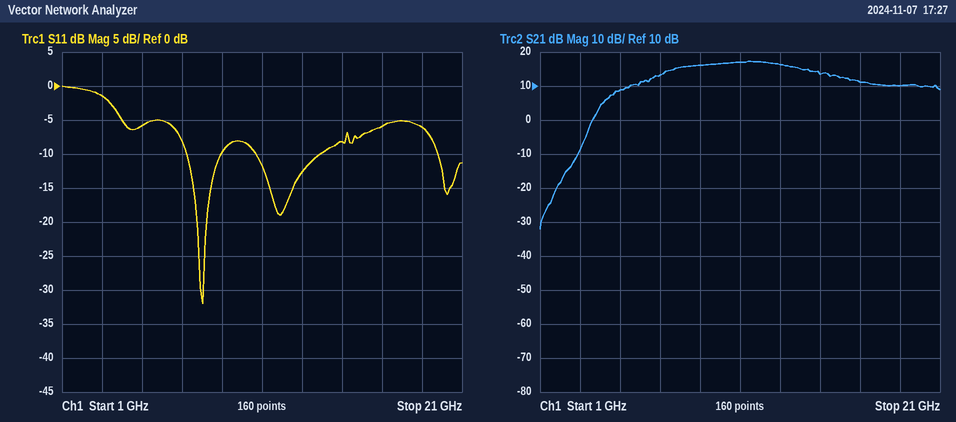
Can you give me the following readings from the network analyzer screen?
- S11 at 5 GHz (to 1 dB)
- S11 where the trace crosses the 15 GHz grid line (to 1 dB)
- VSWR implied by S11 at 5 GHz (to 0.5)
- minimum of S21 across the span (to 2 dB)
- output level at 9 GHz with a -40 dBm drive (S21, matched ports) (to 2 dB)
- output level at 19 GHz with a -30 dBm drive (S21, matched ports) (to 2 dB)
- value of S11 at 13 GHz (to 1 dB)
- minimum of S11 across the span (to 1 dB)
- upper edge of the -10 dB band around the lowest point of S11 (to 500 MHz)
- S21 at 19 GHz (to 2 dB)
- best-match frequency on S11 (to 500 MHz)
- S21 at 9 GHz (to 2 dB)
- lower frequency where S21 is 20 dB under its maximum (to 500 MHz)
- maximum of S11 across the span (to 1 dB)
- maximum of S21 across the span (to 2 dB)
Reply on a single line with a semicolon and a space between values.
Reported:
-6 dB; -8 dB; 3.0; -32 dB; -24 dBm; -20 dBm; -13 dB; -32 dB; 9.0 GHz; 10 dB; 8.0 GHz; 16 dB; 3.5 GHz; 0 dB; 18 dB
